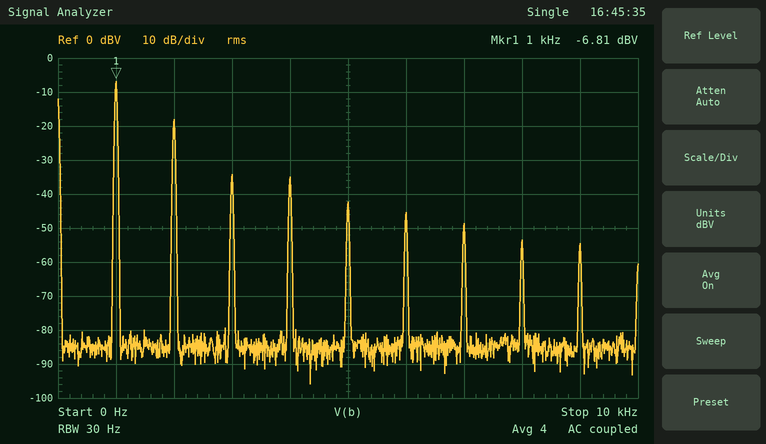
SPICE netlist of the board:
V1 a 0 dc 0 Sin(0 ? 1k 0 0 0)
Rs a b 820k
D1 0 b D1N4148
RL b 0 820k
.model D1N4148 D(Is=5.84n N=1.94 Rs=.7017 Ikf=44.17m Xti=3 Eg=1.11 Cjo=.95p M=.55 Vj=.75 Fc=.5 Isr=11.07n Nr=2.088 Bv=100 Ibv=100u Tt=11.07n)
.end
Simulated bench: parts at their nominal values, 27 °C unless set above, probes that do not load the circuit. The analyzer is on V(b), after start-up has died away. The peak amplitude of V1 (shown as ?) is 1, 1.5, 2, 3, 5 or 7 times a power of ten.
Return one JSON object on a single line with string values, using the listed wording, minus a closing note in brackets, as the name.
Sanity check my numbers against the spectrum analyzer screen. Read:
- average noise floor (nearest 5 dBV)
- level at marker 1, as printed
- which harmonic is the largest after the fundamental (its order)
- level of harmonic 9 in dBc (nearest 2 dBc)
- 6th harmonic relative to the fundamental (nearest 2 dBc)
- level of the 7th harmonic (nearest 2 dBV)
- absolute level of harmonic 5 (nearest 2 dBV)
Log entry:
{"average noise floor": "-85 dBV", "level at marker 1, as printed": "-6.81 dBV", "which harmonic is the largest after the fundamental": "2", "level of harmonic 9 in dBc": "-48 dBc", "6th harmonic relative to the fundamental": "-38 dBc", "level of the 7th harmonic": "-48 dBV", "absolute level of harmonic 5": "-42 dBV"}
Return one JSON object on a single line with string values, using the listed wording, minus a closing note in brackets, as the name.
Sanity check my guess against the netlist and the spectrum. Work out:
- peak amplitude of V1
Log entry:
{"peak amplitude of V1": "2 V"}
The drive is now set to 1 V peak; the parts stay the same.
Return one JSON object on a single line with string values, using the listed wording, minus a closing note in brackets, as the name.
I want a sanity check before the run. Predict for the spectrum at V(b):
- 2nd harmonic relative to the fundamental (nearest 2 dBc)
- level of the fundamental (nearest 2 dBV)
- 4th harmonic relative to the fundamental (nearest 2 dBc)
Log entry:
{"2nd harmonic relative to the fundamental": "-14 dBc", "level of the fundamental": "-12 dBV", "4th harmonic relative to the fundamental": "-34 dBc"}
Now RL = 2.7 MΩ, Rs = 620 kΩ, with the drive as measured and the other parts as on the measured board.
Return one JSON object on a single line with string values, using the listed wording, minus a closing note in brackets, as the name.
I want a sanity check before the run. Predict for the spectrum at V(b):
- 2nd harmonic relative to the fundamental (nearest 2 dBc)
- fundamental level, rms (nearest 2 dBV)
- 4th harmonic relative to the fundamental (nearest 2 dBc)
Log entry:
{"2nd harmonic relative to the fundamental": "-10 dBc", "fundamental level, rms": "-4 dBV", "4th harmonic relative to the fundamental": "-26 dBc"}
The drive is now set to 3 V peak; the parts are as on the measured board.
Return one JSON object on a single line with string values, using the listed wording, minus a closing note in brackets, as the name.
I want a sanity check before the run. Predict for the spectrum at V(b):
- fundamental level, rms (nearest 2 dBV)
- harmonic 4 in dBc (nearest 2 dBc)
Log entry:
{"fundamental level, rms": "-4 dBV", "harmonic 4 in dBc": "-26 dBc"}
